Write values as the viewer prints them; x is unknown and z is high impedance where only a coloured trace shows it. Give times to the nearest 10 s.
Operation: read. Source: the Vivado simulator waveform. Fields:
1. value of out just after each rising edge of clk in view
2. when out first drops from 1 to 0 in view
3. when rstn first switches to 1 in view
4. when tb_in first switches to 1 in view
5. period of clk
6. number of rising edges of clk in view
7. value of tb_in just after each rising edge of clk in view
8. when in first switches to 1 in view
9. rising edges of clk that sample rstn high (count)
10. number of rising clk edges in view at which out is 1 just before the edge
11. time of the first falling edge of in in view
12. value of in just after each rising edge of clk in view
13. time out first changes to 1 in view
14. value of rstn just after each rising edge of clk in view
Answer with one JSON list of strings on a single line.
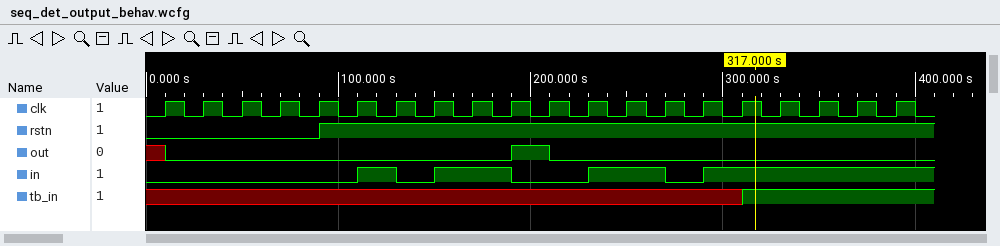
["0 0 0 0 0 0 0 0 0 1 0 0 0 0 0 0 0 0 0 0", "210 s", "90 s", "310 s", "20 s", "20", "x x x x x x x x x x x x x x x 1 1 1 1 1", "110 s", "15", "1", "130 s", "0 0 0 0 0 1 0 1 1 0 0 1 1 0 1 1 1 1 1 1", "190 s", "0 0 0 0 1 1 1 1 1 1 1 1 1 1 1 1 1 1 1 1"]
